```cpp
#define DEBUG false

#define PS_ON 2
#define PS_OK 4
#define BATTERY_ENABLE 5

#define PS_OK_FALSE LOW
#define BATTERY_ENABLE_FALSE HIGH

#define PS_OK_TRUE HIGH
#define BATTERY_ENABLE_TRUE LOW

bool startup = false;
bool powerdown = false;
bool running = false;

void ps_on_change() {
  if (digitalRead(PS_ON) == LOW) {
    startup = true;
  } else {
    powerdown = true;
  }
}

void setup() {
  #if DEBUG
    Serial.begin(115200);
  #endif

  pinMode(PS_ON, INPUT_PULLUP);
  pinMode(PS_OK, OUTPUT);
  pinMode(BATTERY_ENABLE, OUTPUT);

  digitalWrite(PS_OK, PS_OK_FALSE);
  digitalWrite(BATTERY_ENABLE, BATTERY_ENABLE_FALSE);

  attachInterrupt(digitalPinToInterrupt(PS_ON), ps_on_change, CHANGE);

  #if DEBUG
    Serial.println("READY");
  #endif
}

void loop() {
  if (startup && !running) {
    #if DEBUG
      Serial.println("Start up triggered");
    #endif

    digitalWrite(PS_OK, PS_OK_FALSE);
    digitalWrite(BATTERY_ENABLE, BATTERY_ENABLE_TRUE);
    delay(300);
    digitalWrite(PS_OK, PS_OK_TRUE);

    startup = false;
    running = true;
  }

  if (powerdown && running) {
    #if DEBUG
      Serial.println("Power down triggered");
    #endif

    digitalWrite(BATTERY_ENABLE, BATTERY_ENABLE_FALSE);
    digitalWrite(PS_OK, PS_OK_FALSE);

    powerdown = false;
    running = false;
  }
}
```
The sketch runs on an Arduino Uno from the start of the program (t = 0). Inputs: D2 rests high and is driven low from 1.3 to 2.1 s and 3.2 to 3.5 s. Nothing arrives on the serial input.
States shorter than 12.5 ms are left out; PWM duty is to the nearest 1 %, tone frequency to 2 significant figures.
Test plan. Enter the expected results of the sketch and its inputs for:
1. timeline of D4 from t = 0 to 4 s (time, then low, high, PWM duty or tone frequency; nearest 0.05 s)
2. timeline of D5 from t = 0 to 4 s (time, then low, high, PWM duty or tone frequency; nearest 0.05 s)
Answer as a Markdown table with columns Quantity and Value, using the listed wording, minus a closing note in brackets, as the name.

| Quantity | Value |
|---|---|
| timeline of D4 from t = 0 to 4 s | 0 s low; 1.6 s high; 2.1 s low |
| timeline of D5 from t = 0 to 4 s | 0 s high; 1.3 s low; 2.1 s high; 3.2 s low; 3.5 s high |
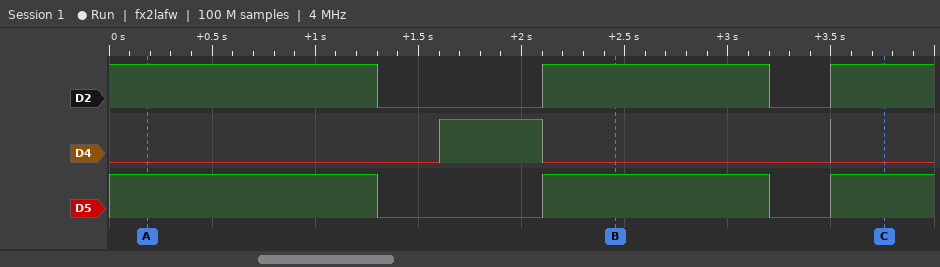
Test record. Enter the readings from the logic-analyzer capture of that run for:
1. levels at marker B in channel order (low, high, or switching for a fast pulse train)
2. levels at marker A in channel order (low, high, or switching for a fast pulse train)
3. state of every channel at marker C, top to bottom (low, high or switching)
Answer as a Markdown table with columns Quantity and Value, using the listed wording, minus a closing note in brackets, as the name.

| Quantity | Value |
|---|---|
| levels at marker B in channel order | D2 high, D4 low, D5 high |
| levels at marker A in channel order | D2 high, D4 low, D5 high |
| state of every channel at marker C, top to bottom | D2 high, D4 low, D5 high |
